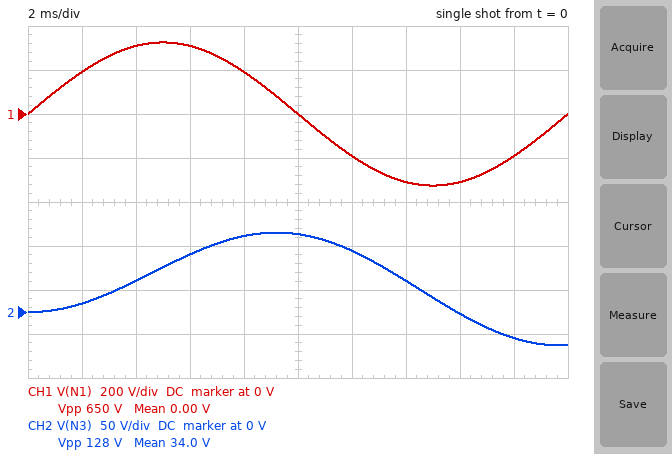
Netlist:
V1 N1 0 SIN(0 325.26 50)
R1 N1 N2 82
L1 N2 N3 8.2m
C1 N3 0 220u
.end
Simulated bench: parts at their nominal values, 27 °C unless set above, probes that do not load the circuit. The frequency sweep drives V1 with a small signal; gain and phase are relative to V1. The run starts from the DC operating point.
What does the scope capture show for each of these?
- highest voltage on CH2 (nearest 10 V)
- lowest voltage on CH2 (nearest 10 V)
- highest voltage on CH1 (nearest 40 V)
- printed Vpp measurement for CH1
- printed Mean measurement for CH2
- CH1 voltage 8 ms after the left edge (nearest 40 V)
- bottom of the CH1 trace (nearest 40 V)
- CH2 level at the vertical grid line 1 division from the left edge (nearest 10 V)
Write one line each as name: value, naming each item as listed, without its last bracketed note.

highest voltage on CH2: 90 V
lowest voltage on CH2: -40 V
highest voltage on CH1: 320 V
printed Vpp measurement for CH1: 650 V
printed Mean measurement for CH2: 34.0 V
CH1 voltage 8 ms after the left edge: 200 V
bottom of the CH1 trace: -320 V
CH2 level at the vertical grid line 1 division from the left edge: 10 V
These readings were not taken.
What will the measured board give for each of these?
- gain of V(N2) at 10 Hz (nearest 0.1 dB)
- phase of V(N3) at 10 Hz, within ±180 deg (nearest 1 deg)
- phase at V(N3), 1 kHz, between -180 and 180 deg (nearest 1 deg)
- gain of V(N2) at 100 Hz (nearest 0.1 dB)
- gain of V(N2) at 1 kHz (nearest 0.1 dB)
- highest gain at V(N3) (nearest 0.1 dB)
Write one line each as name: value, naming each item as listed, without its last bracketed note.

gain of V(N2) at 10 Hz: -3.6 dB
phase of V(N3) at 10 Hz, within ±180 deg: -49 deg
phase at V(N3), 1 kHz, between -180 and 180 deg: -122 deg
gain of V(N2) at 100 Hz: -31.9 dB
gain of V(N2) at 1 kHz: -5.6 dB
highest gain at V(N3): 0 dB
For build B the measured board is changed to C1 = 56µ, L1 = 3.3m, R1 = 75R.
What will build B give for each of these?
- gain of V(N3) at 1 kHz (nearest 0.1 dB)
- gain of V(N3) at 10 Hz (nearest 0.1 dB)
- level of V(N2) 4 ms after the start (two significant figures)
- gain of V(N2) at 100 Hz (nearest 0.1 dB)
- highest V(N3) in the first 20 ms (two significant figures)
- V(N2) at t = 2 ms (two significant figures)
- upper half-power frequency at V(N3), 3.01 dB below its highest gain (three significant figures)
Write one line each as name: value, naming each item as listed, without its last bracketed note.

gain of V(N3) at 1 kHz: -28.7 dB
gain of V(N3) at 10 Hz: -0.3 dB
level of V(N2) 4 ms after the start: 120 V
gain of V(N2) at 100 Hz: -9.6 dB
highest V(N3) in the first 20 ms: 220 V
V(N2) at t = 2 ms: 41 V
upper half-power frequency at V(N3), 3.01 dB below its highest gain: 38.3 Hz
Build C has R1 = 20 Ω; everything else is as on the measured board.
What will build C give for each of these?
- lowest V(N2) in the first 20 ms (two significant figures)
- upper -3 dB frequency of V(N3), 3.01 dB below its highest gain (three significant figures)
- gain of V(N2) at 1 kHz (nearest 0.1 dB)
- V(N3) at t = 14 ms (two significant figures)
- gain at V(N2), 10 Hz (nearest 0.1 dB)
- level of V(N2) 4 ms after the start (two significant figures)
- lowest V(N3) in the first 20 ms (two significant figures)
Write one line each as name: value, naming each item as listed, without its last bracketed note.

lowest V(N2) in the first 20 ms: -160 V
upper -3 dB frequency of V(N3), 3.01 dB below its highest gain: 39.8 Hz
gain of V(N2) at 1 kHz: -0.6 dB
V(N3) at t = 14 ms: -39 V
gain at V(N2), 10 Hz: -0.3 dB
level of V(N2) 4 ms after the start: 110 V
lowest V(N3) in the first 20 ms: -200 V
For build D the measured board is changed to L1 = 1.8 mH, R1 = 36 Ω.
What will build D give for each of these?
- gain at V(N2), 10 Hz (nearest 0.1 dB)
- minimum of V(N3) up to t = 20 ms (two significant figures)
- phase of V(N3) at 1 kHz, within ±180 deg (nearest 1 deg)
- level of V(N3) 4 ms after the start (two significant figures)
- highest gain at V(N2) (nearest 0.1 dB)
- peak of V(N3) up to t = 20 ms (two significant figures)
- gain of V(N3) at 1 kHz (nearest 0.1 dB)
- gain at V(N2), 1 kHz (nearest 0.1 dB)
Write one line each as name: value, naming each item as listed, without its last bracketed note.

gain at V(N2), 10 Hz: -1.0 dB
minimum of V(N3) up to t = 20 ms: -110 V
phase of V(N3) at 1 kHz, within ±180 deg: -106 deg
level of V(N3) 4 ms after the start: 75 V
highest gain at V(N2): 0 dB
peak of V(N3) up to t = 20 ms: 160 V
gain of V(N3) at 1 kHz: -34.3 dB
gain at V(N2), 1 kHz: -11.0 dB
